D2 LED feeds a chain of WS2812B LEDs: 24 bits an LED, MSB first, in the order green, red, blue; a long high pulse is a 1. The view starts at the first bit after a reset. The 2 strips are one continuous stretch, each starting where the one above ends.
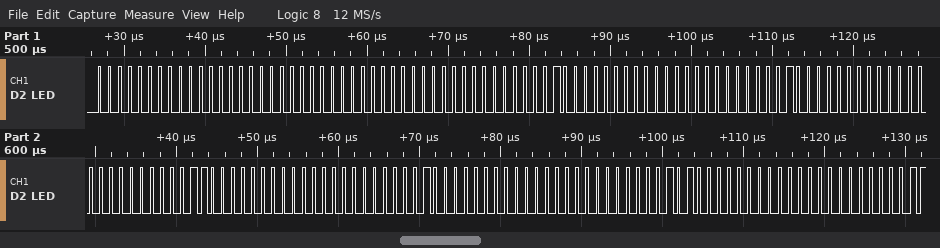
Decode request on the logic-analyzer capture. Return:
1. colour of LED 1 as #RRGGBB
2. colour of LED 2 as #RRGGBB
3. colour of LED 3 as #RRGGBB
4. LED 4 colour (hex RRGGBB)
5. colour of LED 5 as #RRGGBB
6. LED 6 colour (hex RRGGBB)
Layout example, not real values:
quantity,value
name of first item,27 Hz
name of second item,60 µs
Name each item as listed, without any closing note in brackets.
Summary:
quantity,value
colour of LED 1 as #RRGGBB,#000000
colour of LED 2 as #RRGGBB,#000004
colour of LED 3 as #RRGGBB,#000008
LED 4 colour,#00000C
colour of LED 5 as #RRGGBB,#000010
LED 6 colour,#000014
